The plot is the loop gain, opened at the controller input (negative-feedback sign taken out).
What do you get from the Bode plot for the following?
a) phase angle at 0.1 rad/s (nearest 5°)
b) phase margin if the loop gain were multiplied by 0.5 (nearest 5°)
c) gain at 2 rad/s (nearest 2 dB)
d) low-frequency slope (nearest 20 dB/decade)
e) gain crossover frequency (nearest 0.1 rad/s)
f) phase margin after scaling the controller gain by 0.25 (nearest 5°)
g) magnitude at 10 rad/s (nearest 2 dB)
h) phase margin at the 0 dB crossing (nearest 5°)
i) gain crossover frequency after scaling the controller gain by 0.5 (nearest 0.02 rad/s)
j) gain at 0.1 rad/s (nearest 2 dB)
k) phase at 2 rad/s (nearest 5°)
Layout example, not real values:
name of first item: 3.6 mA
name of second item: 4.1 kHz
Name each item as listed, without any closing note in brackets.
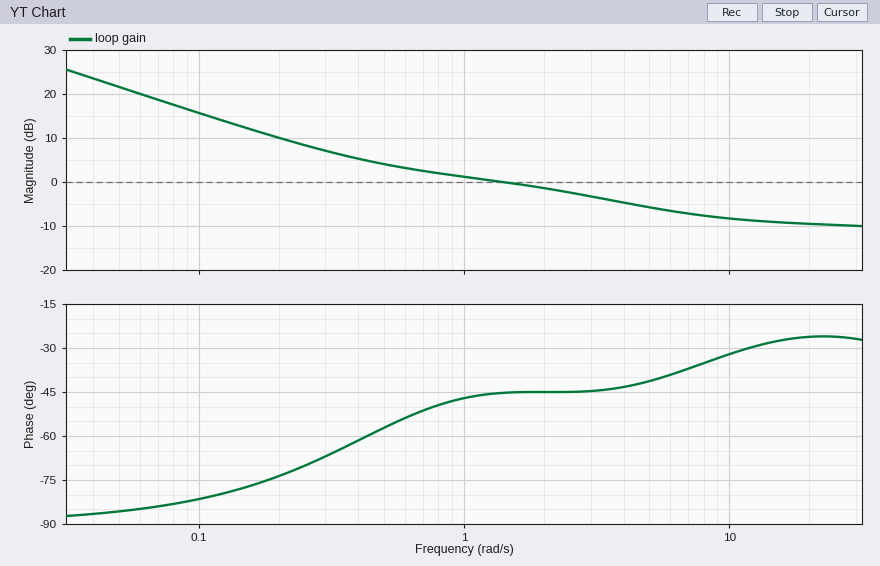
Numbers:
phase angle at 0.1 rad/s: -80°
phase margin if the loop gain were multiplied by 0.5: 115°
gain at 2 rad/s: -2 dB
low-frequency slope: -20 dB/decade
gain crossover frequency: 1.4 rad/s
phase margin after scaling the controller gain by 0.25: 105°
magnitude at 10 rad/s: -8 dB
phase margin at the 0 dB crossing: 135°
gain crossover frequency after scaling the controller gain by 0.5: 0.36 rad/s
gain at 0.1 rad/s: 16 dB
phase at 2 rad/s: -45°
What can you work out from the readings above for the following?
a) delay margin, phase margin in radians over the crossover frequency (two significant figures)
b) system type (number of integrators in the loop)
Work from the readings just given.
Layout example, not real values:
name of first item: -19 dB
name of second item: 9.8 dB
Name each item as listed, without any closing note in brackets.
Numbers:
delay margin, phase margin in radians over the crossover frequency: 1.7 s
system type: 1
